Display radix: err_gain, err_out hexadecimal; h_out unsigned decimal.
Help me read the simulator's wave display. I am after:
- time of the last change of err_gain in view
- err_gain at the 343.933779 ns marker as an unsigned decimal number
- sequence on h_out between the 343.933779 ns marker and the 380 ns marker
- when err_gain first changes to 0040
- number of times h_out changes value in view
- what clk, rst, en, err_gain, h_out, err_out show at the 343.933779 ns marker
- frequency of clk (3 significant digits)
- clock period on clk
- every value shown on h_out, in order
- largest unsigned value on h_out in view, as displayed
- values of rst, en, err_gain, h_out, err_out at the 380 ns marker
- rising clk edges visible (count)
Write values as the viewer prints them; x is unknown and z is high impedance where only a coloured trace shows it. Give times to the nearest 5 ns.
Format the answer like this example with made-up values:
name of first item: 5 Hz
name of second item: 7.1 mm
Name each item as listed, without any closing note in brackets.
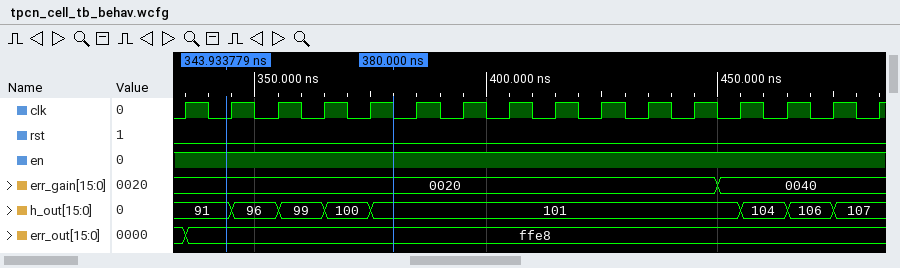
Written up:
time of the last change of err_gain in view: 450 ns
err_gain at the 343.933779 ns marker as an unsigned decimal number: 32
sequence on h_out between the 343.933779 ns marker and the 380 ns marker: 91, 96, 99, 100, 101
when err_gain first changes to 0040: 450 ns
number of times h_out changes value in view: 7
what clk, rst, en, err_gain, h_out, err_out show at the 343.933779 ns marker: clk=0, rst=0, en=1, err_gain=0020, h_out=91, err_out=ffe8
frequency of clk: 100 MHz
clock period on clk: 10 ns
every value shown on h_out, in order: 91, 96, 99, 100, 101, 104, 106, 107
largest unsigned value on h_out in view, as displayed: 107
values of rst, en, err_gain, h_out, err_out at the 380 ns marker: rst=0, en=1, err_gain=0020, h_out=101, err_out=ffe8
rising clk edges visible: 16
